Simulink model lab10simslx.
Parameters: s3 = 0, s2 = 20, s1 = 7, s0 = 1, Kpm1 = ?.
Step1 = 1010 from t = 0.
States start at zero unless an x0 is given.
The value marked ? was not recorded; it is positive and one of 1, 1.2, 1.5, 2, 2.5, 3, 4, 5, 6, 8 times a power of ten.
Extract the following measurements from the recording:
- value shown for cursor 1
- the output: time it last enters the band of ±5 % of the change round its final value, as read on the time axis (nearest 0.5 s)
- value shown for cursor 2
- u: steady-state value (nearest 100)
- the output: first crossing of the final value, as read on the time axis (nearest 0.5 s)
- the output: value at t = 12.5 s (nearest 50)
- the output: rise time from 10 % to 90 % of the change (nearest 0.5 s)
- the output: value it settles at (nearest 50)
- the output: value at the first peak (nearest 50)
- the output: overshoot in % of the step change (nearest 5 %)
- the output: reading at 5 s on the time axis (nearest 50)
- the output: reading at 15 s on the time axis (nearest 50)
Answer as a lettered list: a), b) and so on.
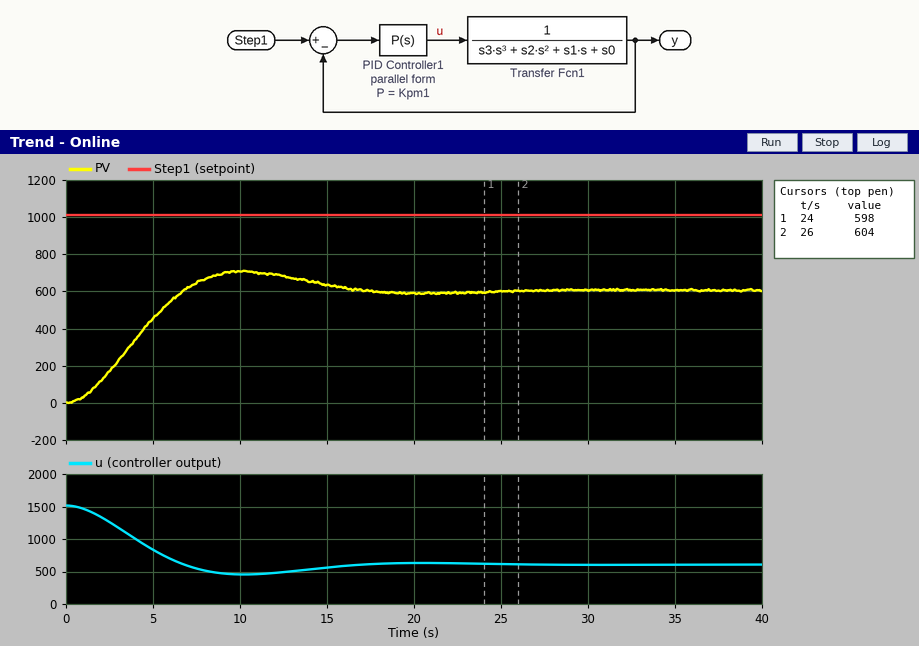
a) 598
b) 15.0 s
c) 604
d) 600
e) 7.0 s
f) 700
g) 4.5 s
h) 600
i) 700
j) 15 %
k) 450
l) 650
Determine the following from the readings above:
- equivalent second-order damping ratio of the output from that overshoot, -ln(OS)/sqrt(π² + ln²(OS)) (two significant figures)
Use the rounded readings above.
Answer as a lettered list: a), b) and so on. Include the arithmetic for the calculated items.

a) ln(0.15) = -1.897; 1.897 / sqrt(9.870 + 3.599) = 0.52
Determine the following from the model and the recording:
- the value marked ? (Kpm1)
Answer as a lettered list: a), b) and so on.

a) 1.5
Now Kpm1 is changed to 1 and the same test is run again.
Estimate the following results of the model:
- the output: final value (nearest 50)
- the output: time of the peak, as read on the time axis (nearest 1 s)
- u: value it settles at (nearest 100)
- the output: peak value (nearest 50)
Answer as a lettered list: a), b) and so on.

a) 500
b) 12 s
c) 500
d) 550
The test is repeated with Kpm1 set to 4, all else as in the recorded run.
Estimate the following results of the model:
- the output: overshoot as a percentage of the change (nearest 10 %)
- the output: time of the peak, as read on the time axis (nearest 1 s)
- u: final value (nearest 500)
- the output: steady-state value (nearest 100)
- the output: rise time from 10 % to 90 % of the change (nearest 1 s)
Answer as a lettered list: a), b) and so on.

a) 30 %
b) 7 s
c) 1000
d) 800
e) 3 s
